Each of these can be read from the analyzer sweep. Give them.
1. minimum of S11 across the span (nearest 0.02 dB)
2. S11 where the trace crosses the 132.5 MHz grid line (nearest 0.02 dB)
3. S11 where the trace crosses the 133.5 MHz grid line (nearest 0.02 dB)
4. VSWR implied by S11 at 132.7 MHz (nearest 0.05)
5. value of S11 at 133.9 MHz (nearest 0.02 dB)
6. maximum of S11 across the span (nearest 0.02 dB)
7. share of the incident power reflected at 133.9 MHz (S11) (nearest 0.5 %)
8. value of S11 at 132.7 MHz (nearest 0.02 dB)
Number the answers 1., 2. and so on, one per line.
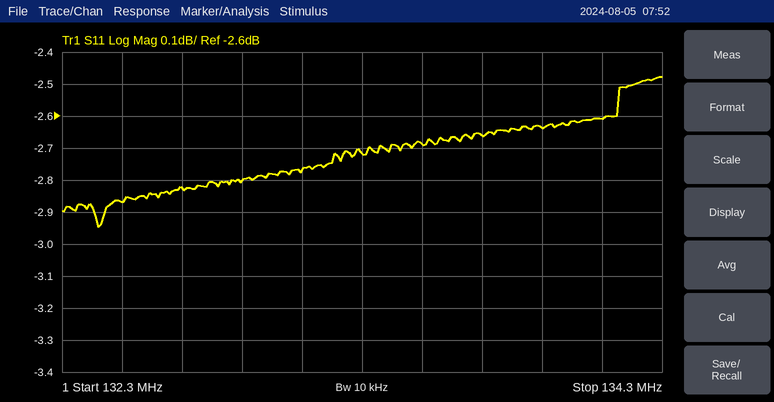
1. -2.94 dB
2. -2.86 dB
3. -2.68 dB
4. 6.20
5. -2.64 dB
6. -2.48 dB
7. 54.5 %
8. -2.82 dB
